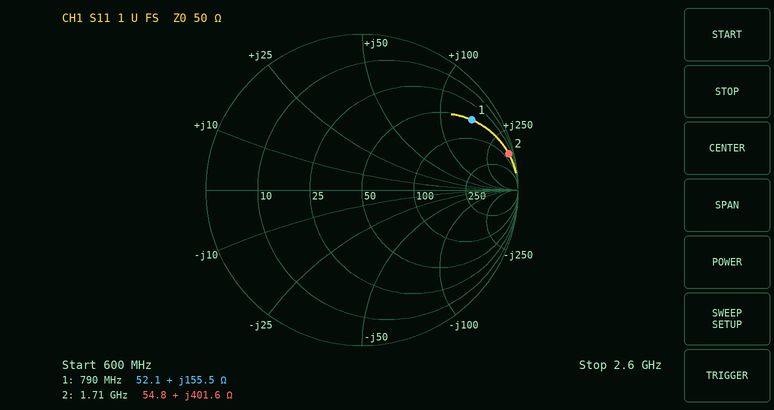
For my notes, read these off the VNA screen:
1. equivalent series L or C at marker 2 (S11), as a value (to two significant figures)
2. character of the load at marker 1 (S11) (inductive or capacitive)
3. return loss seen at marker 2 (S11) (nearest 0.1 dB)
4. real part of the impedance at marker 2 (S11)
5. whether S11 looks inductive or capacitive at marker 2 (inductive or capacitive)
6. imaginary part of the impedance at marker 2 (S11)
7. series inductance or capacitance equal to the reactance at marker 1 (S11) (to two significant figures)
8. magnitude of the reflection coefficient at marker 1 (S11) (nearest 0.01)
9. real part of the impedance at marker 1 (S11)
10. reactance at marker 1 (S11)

37 nH
inductive
0.3 dB
54.8 Ω
inductive
+401.6 Ω
31 nH
0.84
52.1 Ω
+155.5 Ω
